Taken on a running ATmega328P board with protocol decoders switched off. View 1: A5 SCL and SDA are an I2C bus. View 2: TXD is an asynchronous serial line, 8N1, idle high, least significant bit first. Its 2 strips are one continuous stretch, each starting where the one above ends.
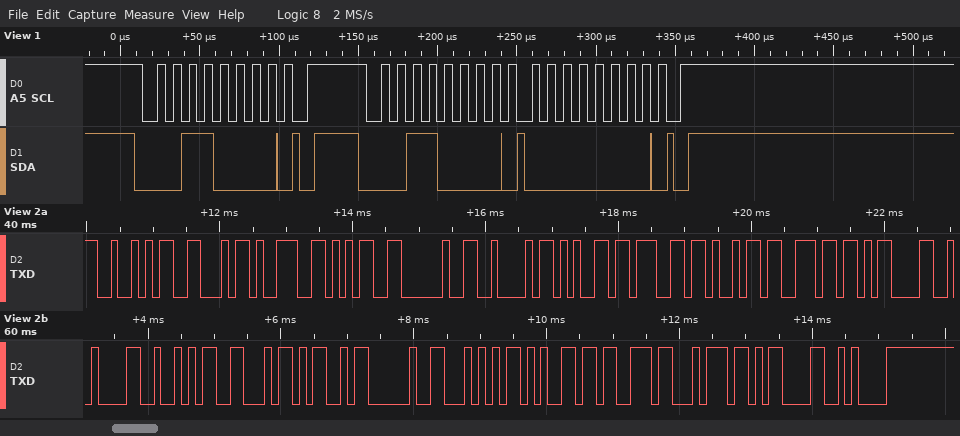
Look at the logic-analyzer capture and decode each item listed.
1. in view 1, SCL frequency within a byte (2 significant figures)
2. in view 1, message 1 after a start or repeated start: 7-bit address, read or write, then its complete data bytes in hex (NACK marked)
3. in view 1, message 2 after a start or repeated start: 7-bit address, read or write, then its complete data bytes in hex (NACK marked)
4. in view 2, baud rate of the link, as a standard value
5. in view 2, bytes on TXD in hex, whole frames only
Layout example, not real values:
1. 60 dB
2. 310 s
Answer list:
1. 100 kHz
2. 0x18 write
3. 0x18 write: 00
4. 9600 baud
5. 0x52 0x46 0x39 0x35 0x20 0x42 0x65 0x67 0x69 0x6E 0x0D 0x0A 0x52 0x46 0x4D 0x20 0x54 0x65 0x73 0x74 0x0D 0x0A
